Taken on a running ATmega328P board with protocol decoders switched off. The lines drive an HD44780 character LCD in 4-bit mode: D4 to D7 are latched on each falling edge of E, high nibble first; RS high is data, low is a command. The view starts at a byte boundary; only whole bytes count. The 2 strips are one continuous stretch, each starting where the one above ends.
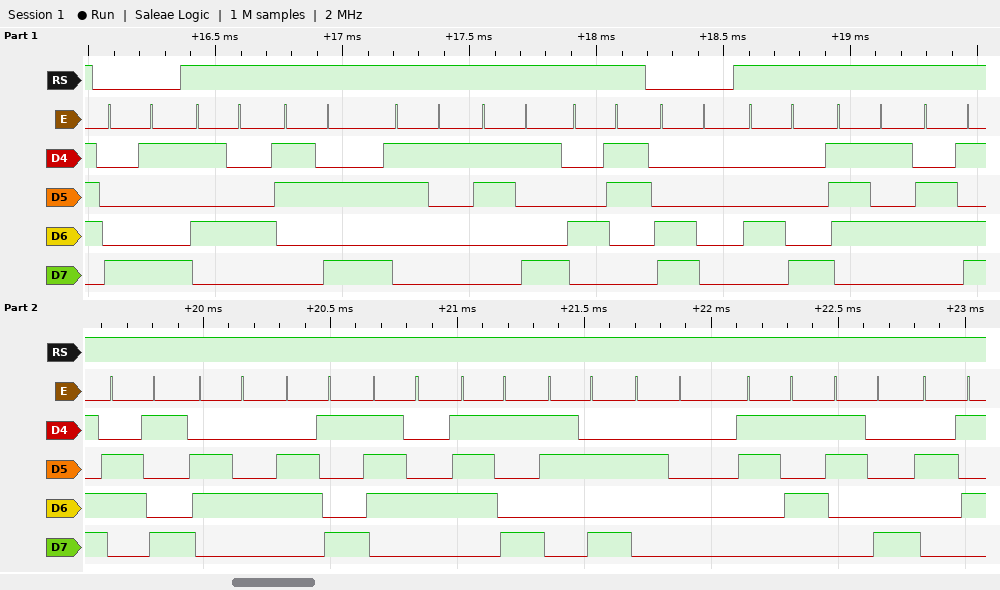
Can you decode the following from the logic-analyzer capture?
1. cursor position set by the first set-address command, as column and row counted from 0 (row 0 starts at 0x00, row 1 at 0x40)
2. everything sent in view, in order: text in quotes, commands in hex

column 9, row 0
0x89 "T:19C" 0xC0 "Humidity: 58%"
